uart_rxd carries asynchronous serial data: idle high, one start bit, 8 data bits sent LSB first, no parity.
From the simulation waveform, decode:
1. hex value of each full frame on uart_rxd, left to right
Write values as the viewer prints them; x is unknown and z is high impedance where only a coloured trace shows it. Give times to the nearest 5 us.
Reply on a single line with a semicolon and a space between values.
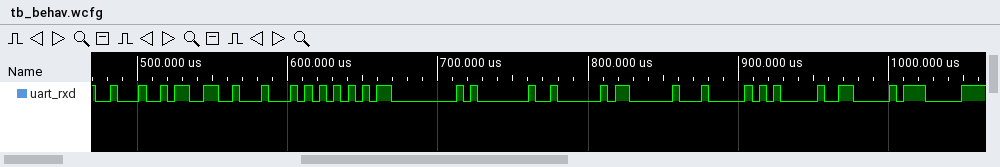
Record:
22, 33, 44, 55, 00, 01, 02, 03, 04, 05, 06, 07
